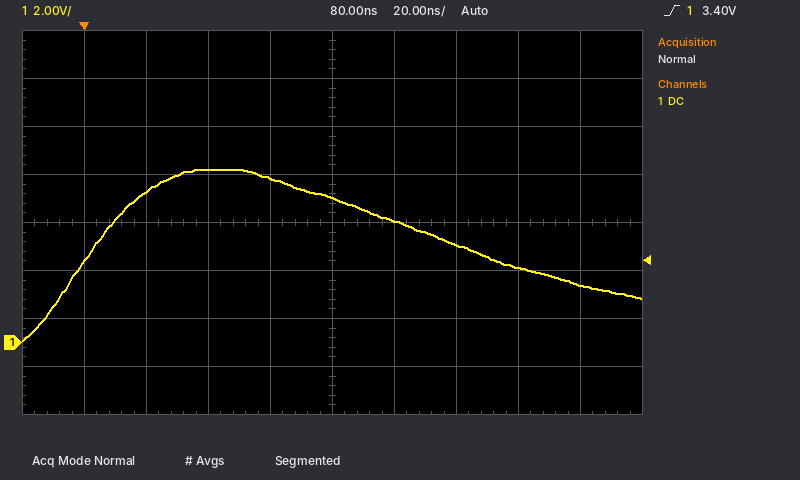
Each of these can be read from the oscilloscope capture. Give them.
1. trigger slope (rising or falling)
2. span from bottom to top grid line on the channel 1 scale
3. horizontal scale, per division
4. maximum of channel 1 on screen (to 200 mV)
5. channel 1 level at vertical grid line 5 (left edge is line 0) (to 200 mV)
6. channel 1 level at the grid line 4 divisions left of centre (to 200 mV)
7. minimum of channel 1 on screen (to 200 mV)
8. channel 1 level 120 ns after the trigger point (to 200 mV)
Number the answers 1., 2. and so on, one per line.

1. rising
2. 16 V
3. 20 ns
4. 7.2 V
5. 6.0 V
6. 3.4 V
7. 0.0 V
8. 4.0 V
